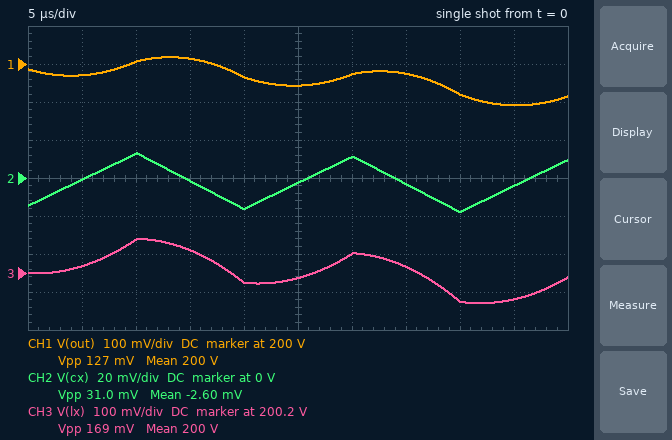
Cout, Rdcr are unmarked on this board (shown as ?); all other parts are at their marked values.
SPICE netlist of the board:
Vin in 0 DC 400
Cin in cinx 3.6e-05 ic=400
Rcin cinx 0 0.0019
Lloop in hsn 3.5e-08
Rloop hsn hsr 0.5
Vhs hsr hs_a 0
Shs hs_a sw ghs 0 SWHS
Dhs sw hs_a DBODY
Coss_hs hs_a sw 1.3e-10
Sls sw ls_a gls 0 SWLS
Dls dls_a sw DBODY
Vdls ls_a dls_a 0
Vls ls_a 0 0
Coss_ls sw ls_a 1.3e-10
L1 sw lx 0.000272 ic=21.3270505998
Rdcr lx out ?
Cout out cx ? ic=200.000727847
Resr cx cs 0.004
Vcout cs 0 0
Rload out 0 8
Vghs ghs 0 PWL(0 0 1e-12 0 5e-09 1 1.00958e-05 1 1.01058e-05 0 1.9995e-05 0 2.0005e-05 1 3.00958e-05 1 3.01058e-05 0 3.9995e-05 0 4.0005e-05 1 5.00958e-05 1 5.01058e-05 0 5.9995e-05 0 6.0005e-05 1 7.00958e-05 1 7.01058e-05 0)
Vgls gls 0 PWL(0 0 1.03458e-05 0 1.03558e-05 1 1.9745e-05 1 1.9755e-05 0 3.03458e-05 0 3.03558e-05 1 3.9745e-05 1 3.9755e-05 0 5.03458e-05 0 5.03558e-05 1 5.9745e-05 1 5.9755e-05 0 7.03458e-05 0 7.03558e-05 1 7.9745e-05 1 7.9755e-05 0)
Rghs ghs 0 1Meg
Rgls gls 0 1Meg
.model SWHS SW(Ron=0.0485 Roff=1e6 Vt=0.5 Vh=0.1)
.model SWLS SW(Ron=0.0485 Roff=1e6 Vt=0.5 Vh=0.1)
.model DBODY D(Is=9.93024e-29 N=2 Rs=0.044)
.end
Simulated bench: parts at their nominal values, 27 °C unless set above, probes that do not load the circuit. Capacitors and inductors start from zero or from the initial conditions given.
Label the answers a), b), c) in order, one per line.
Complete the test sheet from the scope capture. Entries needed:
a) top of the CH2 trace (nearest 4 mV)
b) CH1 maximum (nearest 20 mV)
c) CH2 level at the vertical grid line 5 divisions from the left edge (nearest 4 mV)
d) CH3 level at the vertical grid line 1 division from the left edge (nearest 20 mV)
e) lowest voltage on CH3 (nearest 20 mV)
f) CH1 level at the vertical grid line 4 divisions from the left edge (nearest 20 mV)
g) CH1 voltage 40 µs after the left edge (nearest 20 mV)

a) 12 mV
b) 200.02 V
c) -4 mV
d) 200.22 V
e) 200.12 V
f) 199.96 V
g) 199.92 V
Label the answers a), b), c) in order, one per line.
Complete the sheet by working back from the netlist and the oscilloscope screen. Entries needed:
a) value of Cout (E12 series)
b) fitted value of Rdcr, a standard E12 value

a) 330 µF
b) 0.01 Ω
